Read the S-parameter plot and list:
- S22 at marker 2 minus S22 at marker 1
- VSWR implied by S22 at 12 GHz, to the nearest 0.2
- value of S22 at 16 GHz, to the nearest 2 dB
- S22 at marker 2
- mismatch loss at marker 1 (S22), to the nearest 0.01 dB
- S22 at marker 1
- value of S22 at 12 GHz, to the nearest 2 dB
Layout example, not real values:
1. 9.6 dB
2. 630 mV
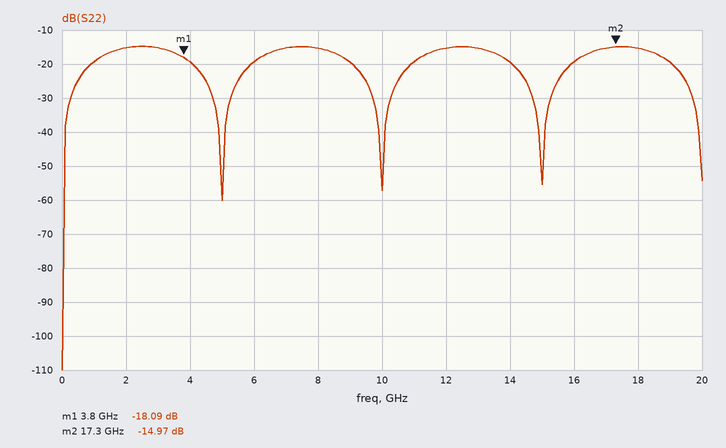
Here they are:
1. 3.12 dB
2. 1.4
3. -20 dB
4. -14.97 dB
5. 0.07 dB
6. -18.09 dB
7. -16 dB
